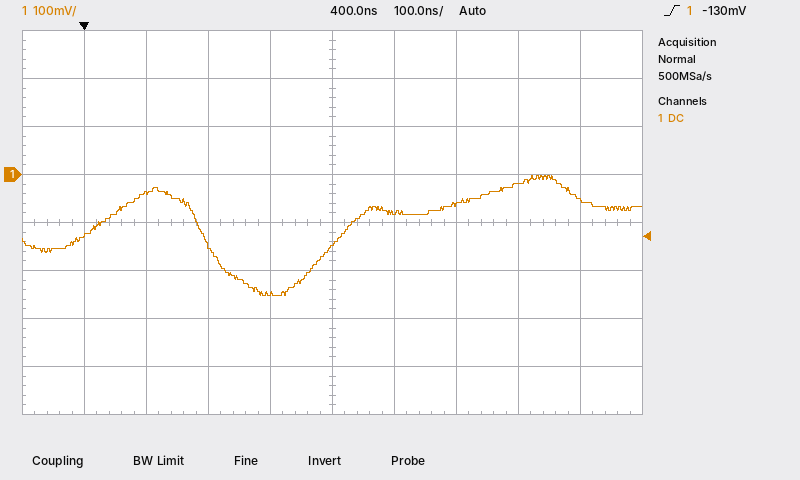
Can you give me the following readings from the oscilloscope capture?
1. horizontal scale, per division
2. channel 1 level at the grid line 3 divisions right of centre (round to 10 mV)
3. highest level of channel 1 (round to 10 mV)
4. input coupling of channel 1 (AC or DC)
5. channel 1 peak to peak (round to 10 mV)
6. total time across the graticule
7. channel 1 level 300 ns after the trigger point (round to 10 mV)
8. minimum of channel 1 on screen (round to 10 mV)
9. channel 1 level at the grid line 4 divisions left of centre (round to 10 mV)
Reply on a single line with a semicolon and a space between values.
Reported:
100 ns; -20 mV; 0 mV; DC; 250 mV; 1 µs; -250 mV; -250 mV; -130 mV
